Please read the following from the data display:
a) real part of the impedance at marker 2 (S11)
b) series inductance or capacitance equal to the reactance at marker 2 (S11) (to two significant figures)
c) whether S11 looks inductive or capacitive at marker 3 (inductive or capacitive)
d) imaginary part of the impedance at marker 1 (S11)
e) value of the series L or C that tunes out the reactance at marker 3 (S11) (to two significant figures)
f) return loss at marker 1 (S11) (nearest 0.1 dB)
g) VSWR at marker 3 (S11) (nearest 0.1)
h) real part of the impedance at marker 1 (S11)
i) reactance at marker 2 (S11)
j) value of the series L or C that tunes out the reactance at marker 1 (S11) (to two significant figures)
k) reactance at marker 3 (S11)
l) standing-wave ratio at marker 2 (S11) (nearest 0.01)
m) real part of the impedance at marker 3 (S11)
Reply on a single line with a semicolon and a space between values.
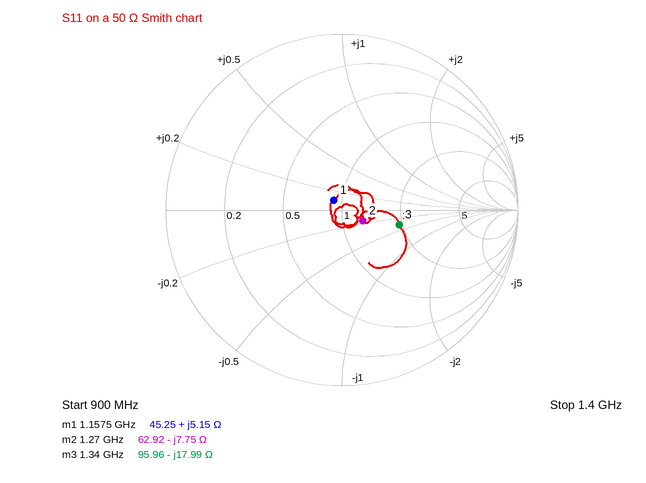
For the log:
62.92 Ω; 16 pF; capacitive; +5.15 Ω; 2.1 nH; 22.7 dB; 2.0; 45.25 Ω; -7.75 Ω; 27 pF; -17.99 Ω; 1.31; 95.96 Ω
